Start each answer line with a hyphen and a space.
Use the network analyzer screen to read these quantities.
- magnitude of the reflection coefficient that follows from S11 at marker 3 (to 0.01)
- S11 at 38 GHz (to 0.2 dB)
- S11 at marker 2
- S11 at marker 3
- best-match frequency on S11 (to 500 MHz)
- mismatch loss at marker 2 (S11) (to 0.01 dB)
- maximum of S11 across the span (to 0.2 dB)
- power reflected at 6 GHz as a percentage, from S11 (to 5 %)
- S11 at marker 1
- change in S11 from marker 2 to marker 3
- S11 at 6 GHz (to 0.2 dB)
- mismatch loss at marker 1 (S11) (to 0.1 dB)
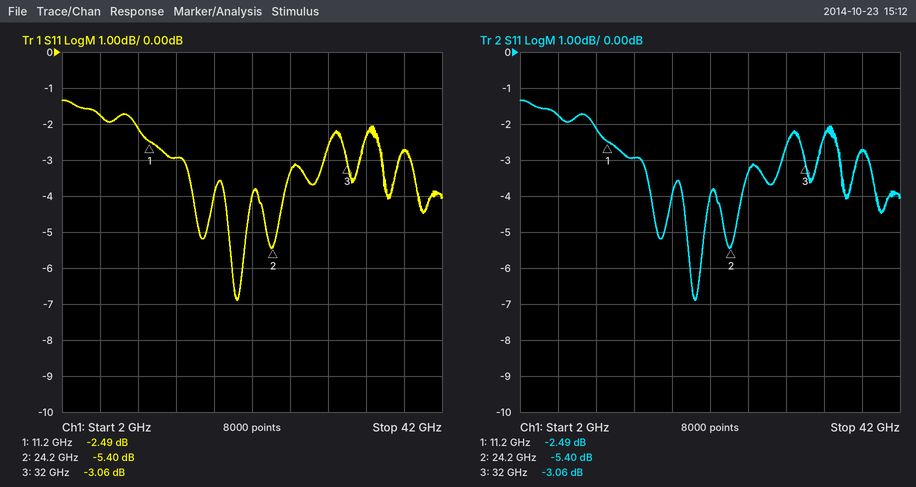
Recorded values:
- 0.70
- -2.8 dB
- -5.40 dB
- -3.06 dB
- 20.5 GHz
- 1.48 dB
- -1.4 dB
- 65 %
- -2.49 dB
- 2.34 dB
- -1.8 dB
- 3.6 dB
